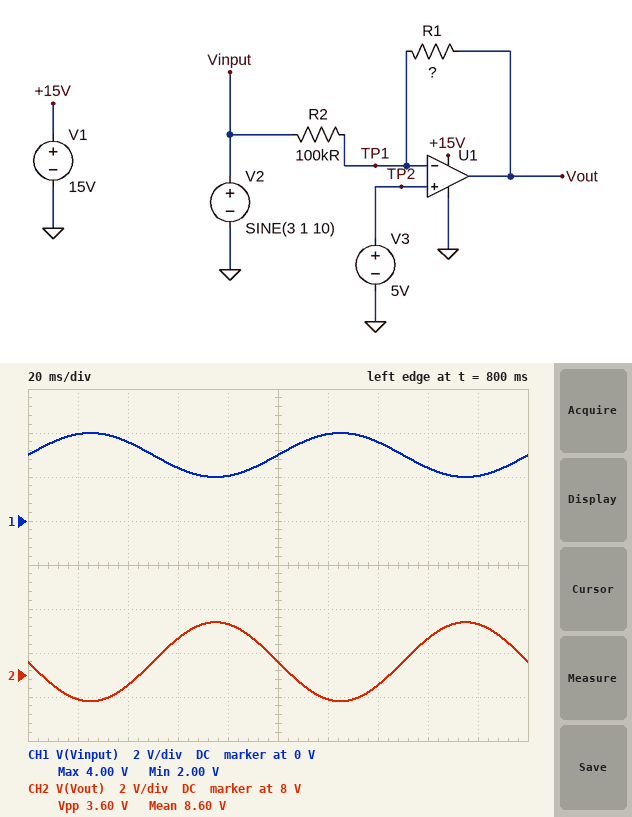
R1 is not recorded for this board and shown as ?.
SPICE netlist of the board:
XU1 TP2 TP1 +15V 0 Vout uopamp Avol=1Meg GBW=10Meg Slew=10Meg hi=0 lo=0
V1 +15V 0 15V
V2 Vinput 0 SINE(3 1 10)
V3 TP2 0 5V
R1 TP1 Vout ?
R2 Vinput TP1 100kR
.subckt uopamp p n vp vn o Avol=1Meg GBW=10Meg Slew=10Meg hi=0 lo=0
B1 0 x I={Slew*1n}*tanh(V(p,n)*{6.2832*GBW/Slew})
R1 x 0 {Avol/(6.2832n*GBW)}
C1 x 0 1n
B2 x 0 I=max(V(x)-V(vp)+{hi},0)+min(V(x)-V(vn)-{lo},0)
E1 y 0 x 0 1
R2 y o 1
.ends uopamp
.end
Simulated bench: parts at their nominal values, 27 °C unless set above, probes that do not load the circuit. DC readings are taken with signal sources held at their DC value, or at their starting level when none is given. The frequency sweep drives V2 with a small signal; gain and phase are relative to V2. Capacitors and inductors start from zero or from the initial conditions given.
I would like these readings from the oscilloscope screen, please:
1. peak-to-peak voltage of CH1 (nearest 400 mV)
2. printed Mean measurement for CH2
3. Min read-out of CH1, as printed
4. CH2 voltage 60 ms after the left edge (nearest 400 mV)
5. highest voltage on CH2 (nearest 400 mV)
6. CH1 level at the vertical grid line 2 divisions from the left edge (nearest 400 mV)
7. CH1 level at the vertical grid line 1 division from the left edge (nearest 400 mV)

2.0 V
8.60 V
2.00 V
9.6 V
10.4 V
3.6 V
4.0 V
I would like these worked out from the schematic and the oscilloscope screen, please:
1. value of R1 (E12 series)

180 kΩ
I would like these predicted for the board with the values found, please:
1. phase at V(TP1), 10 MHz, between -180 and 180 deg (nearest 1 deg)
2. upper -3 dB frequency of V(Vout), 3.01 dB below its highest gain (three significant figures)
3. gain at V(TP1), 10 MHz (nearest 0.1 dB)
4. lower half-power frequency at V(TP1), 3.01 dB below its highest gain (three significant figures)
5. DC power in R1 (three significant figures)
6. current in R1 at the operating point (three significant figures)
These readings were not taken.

20 deg
3.57 MHz
-4.4 dB
3.57 MHz
72.0 µW
20.0 µA
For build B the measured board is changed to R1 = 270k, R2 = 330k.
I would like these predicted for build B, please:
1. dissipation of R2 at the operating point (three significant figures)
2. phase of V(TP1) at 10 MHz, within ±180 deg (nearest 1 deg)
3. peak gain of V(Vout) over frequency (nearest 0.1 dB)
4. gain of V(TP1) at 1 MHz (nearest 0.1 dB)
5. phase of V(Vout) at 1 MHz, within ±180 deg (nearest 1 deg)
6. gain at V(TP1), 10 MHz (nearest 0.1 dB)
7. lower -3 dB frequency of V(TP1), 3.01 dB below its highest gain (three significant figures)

12.1 µW
29 deg
-1.7 dB
-21.9 dB
170 deg
-8.1 dB
5.50 MHz
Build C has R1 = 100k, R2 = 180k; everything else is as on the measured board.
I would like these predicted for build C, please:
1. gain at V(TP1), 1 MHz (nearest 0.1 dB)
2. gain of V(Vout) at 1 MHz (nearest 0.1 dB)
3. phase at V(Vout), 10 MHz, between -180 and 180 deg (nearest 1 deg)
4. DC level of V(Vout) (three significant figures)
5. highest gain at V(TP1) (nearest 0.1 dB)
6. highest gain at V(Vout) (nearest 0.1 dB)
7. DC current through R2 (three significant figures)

-25.2 dB
-5.2 dB
123 deg
6.11 V
-8.9 dB
-5.1 dB
11.1 µA
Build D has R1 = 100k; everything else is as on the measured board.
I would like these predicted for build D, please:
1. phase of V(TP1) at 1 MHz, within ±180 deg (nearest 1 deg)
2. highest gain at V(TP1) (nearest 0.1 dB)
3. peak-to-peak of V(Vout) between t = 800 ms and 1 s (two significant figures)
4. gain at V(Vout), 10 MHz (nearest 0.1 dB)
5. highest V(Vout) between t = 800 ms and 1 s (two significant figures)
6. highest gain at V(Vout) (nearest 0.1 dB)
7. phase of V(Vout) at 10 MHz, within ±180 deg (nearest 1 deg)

79 deg
-6.0 dB
2.0 V
-7.0 dB
8.0 V
0 dB
117 deg
